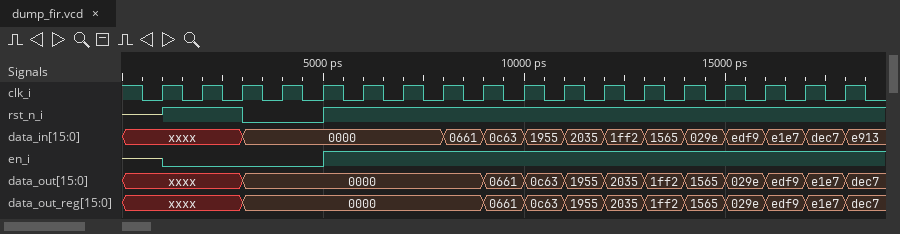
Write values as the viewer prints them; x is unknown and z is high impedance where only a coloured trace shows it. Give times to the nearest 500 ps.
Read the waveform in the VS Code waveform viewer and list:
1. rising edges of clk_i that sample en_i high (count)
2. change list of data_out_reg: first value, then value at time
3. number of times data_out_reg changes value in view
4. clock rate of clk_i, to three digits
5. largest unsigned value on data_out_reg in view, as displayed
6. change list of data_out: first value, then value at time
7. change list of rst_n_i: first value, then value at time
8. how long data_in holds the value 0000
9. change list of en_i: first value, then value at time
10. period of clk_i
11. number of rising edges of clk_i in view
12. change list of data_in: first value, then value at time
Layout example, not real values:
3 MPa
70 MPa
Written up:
13
xxxx, 0000 at 3000 ps, 0661 at 9000 ps, 0c63 at 10000 ps, 1955 at 11000 ps, 2035 at 12000 ps, 1ff2 at 13000 ps, 1565 at 14000 ps, 029e at 15000 ps, edf9 at 16000 ps, e1e7 at 17000 ps, dec7 at 18000 ps
11
1.00 GHz
edf9
xxxx, 0000 at 3000 ps, 0661 at 9000 ps, 0c63 at 10000 ps, 1955 at 11000 ps, 2035 at 12000 ps, 1ff2 at 13000 ps, 1565 at 14000 ps, 029e at 15000 ps, edf9 at 16000 ps, e1e7 at 17000 ps, dec7 at 18000 ps
z, 1 at 1000 ps, 0 at 3000 ps, 1 at 5000 ps
5000 ps
z, 0 at 1000 ps, 1 at 5000 ps
1000 ps
18
xxxx, 0000 at 3000 ps, 0661 at 8000 ps, 0c63 at 9000 ps, 1955 at 10000 ps, 2035 at 11000 ps, 1ff2 at 12000 ps, 1565 at 13000 ps, 029e at 14000 ps, edf9 at 15000 ps, e1e7 at 16000 ps, dec7 at 17000 ps, e913 at 18000 ps
